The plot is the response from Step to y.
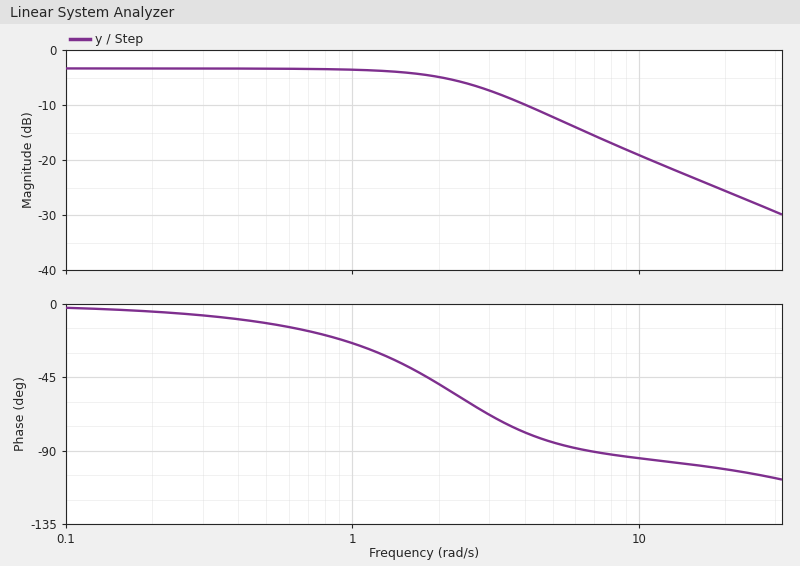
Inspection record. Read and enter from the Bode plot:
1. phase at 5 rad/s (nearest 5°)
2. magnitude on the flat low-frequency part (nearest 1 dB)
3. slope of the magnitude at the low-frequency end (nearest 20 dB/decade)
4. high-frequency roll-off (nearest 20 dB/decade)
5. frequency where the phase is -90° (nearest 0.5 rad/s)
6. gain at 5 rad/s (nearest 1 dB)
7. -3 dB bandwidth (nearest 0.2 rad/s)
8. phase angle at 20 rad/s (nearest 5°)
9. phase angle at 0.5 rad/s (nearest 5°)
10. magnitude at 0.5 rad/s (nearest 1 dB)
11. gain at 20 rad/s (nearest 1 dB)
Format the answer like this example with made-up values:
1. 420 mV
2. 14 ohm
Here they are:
1. -85°
2. -3 dB
3. 0 dB/decade
4. -20 dB/decade
5. 6.5 rad/s
6. -12 dB
7. 2.6 rad/s
8. -100°
9. -10°
10. -3 dB
11. -26 dB
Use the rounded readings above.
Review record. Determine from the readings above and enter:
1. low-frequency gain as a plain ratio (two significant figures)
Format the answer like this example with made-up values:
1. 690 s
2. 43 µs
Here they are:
1. 0.71
